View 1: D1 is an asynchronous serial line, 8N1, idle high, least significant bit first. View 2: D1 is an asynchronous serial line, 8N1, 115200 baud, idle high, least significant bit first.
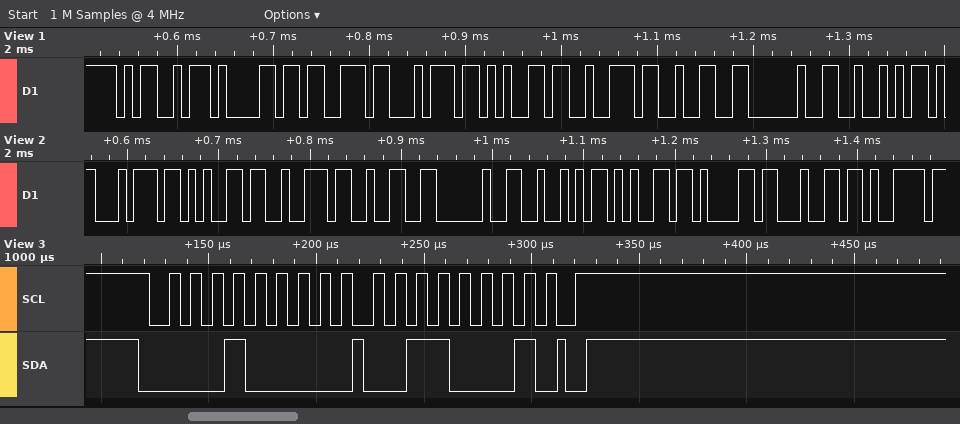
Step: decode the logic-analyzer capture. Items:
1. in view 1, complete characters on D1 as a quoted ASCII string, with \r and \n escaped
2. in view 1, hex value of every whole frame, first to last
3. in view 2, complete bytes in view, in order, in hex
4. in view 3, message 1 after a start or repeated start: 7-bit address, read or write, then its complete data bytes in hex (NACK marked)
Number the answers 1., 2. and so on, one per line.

1. "Master2 R"
2. 4D 61 73 74 65 72 32 20 52
3. 74 65 72 32 20 52 65 61 64 79
4. 0x08 write: 31
